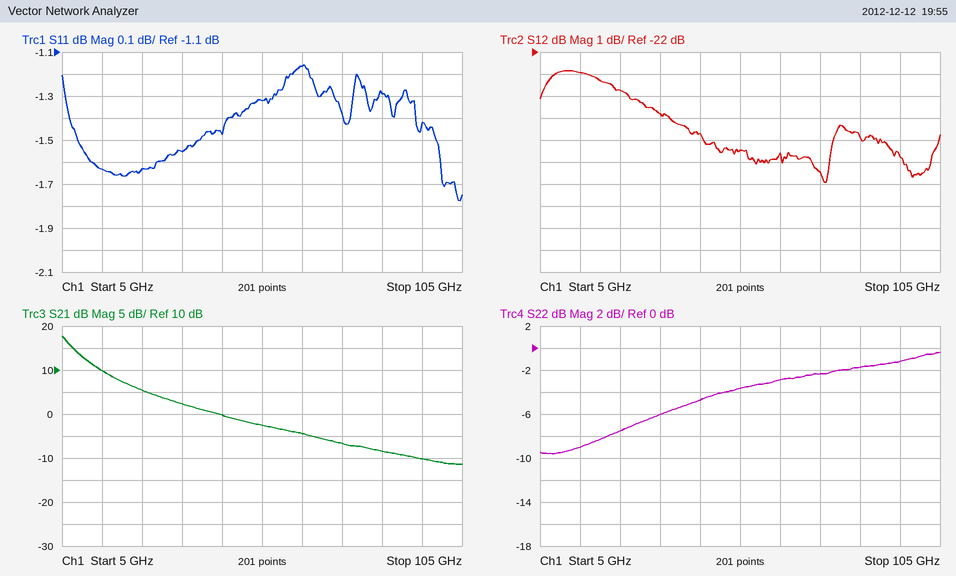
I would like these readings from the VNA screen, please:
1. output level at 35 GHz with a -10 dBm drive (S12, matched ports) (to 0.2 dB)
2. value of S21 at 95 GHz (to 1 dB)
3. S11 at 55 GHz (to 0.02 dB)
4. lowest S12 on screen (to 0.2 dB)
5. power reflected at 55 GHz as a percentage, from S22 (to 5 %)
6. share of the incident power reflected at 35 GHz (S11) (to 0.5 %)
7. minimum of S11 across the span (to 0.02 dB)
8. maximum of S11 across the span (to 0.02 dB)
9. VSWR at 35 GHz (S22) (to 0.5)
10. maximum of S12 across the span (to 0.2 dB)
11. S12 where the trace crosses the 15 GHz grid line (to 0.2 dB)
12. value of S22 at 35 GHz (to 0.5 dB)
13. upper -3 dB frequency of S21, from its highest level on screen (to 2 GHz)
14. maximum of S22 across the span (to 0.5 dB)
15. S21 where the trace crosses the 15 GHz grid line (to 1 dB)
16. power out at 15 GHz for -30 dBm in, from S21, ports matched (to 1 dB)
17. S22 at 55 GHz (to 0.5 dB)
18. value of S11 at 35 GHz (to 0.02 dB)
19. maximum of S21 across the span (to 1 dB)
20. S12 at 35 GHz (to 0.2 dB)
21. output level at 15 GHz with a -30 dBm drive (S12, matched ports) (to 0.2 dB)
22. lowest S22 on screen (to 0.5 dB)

-34.8 dBm
-10 dB
-1.32 dB
-28.0 dB
45 %
70.0 %
-1.78 dB
-1.16 dB
3.0
-22.8 dB
-23.0 dB
-6.0 dB
8 GHz
-0.5 dB
10 dB
-20 dBm
-3.5 dB
-1.56 dB
18 dB
-24.8 dB
-53.0 dBm
-9.5 dB
